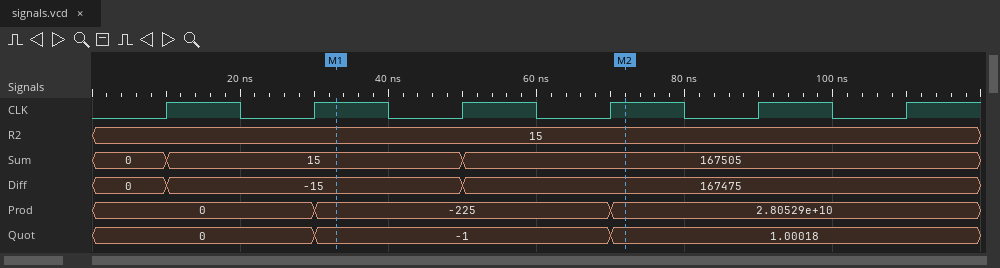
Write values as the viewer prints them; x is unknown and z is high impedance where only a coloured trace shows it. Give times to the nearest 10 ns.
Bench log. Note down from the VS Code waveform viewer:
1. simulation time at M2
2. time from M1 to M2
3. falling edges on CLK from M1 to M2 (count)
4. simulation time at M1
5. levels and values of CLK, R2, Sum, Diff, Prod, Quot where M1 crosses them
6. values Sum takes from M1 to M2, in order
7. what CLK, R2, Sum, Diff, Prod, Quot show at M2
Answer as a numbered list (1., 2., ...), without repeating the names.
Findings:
1. 70 ns
2. 40 ns
3. 2
4. 30 ns
5. CLK=1, R2=15, Sum=15, Diff=-15, Prod=-225, Quot=-1
6. 15, 167505
7. CLK=1, R2=15, Sum=167505, Diff=167475, Prod=2.80529e+10, Quot=1.00018
